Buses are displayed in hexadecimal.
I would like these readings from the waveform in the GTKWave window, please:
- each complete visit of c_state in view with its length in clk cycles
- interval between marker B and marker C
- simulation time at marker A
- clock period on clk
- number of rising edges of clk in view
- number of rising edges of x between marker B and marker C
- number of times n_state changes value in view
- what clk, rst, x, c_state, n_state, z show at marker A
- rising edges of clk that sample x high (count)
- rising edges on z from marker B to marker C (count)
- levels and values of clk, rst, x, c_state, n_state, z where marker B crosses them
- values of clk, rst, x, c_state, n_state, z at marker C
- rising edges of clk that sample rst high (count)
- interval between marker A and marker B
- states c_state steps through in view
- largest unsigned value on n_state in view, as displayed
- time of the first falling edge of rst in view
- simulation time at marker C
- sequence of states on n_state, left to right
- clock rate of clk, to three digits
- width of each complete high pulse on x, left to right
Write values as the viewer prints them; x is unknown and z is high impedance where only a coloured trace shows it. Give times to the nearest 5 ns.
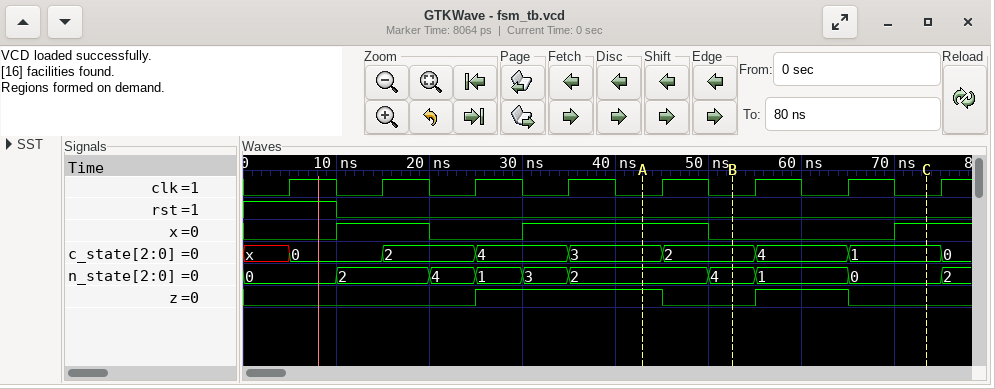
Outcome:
0: 1, 2: 1, 4: 1, 3: 1, 2: 1, 4: 1, 1: 1
20 ns
45 ns
10 ns
8
1
9
clk=0, rst=0, x=1, c_state=3, n_state=2, z=1
4
1
clk=0, rst=0, x=0, c_state=2, n_state=4, z=0
clk=0, rst=0, x=1, c_state=1, n_state=0, z=0
1
10 ns
x, 0, 2, 4, 3, 2, 4, 1, 0
4
10 ns
75 ns
0, 2, 4, 1, 3, 2, 4, 1, 0, 2
100 MHz
10 ns, 20 ns
